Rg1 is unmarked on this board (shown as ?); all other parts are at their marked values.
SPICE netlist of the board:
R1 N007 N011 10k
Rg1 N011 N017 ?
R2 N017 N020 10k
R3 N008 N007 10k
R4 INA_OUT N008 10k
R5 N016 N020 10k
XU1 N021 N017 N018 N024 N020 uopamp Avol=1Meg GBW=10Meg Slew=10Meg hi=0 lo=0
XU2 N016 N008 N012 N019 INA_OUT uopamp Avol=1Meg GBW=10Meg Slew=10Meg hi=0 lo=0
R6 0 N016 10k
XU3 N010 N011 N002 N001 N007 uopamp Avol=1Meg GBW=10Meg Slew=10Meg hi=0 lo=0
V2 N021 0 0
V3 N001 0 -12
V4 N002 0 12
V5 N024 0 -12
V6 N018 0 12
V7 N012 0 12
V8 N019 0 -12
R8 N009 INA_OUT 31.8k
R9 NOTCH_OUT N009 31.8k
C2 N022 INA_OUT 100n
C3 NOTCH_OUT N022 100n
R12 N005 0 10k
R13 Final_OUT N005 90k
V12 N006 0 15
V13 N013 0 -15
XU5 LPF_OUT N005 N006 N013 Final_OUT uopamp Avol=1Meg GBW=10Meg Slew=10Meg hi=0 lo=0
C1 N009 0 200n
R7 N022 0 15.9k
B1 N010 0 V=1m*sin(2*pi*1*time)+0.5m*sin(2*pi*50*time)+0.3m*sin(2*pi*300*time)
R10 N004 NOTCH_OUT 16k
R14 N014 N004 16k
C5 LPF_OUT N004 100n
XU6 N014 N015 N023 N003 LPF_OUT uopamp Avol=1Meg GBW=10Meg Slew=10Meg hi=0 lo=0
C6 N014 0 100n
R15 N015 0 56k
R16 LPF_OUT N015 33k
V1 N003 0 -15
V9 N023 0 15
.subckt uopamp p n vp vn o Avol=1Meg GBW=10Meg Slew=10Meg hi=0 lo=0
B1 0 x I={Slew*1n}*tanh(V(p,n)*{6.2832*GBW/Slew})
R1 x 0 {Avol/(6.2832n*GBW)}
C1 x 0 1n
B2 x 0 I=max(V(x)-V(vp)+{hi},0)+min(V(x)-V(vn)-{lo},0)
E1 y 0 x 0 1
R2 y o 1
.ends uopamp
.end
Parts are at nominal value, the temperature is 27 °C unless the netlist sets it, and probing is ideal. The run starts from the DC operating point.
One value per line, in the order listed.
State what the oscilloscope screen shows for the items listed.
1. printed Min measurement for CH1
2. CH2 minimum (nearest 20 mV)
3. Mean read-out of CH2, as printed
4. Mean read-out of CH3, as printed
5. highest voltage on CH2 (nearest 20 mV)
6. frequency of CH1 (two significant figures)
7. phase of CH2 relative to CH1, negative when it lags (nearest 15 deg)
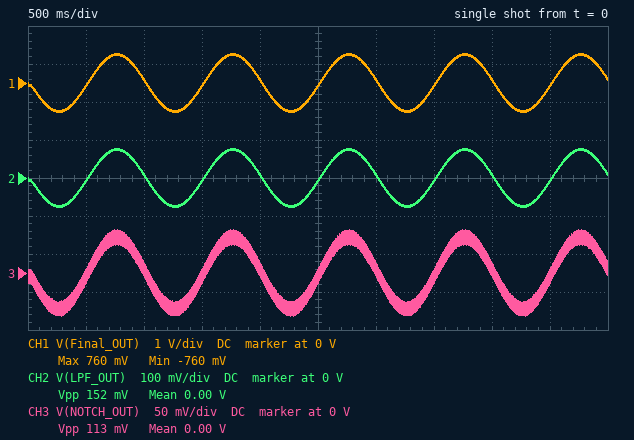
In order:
-760 mV
-80 mV
0.00 V
0.00 V
80 mV
1.0 Hz
0 deg
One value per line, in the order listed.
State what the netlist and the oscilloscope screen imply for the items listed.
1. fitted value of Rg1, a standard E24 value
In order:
430 Ω
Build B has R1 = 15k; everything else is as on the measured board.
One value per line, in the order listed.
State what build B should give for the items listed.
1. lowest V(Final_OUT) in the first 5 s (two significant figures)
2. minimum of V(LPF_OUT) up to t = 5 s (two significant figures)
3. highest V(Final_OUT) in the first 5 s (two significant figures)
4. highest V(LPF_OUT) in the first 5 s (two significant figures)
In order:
-950 mV
-95 mV
950 mV
95 mV
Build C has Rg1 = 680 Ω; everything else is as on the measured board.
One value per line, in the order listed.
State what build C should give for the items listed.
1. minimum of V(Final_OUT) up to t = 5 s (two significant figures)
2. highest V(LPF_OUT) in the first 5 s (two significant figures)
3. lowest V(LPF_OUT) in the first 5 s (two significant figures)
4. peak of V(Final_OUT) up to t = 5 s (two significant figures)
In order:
-490 mV
49 mV
-49 mV
490 mV
